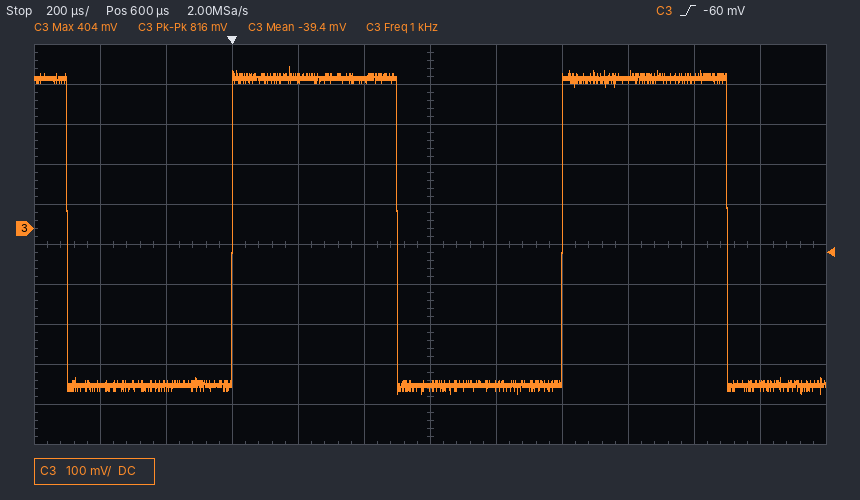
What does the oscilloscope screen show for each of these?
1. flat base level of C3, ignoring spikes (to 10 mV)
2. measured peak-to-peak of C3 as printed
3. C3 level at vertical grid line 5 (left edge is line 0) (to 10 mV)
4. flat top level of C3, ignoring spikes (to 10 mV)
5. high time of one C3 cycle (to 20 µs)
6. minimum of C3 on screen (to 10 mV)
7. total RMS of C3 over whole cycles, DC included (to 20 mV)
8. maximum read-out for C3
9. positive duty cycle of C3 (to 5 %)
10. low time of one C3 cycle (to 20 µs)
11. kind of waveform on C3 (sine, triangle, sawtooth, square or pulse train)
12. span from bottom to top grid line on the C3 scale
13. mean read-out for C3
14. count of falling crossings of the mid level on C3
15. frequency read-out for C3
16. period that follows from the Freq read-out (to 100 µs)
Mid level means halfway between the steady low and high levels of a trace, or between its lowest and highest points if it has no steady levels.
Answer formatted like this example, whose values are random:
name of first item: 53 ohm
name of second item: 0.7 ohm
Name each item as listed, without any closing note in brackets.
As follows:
flat base level of C3, ignoring spikes: -390 mV
measured peak-to-peak of C3 as printed: 816 mV
C3 level at vertical grid line 5 (left edge is line 0): 370 mV
flat top level of C3, ignoring spikes: 380 mV
high time of one C3 cycle: 500 µs
minimum of C3 on screen: -410 mV
total RMS of C3 over whole cycles, DC included: 380 mV
maximum read-out for C3: 404 mV
positive duty cycle of C3: 50 %
low time of one C3 cycle: 500 µs
kind of waveform on C3: square
span from bottom to top grid line on the C3 scale: 1 V
mean read-out for C3: -39.4 mV
count of falling crossings of the mid level on C3: 3
frequency read-out for C3: 1 kHz
period that follows from the Freq read-out: 1.0 ms
